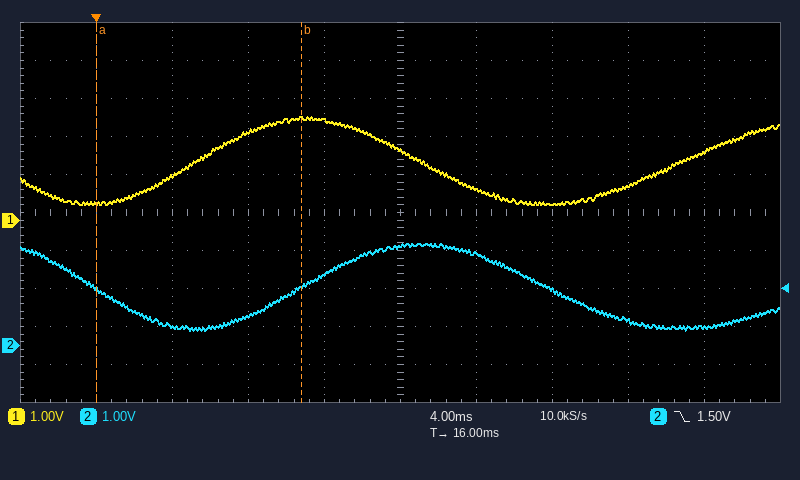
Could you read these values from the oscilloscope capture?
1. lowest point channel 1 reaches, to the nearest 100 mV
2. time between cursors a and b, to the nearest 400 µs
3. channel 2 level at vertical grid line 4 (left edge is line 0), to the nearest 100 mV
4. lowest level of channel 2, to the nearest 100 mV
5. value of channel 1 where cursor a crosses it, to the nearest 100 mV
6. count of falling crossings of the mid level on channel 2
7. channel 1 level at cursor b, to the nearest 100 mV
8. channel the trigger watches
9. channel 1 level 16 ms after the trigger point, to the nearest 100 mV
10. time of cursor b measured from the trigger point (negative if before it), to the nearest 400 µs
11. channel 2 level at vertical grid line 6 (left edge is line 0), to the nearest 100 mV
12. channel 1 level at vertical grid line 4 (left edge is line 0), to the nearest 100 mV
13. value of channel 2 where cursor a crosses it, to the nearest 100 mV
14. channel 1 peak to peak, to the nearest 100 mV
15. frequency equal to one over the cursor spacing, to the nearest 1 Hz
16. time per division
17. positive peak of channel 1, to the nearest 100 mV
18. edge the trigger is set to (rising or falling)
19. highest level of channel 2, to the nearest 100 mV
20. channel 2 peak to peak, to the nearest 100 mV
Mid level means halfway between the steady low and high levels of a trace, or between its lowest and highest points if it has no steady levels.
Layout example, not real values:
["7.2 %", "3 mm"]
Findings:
["400 mV", "10.8 ms", "1.9 V", "400 mV", "400 mV", "2", "2.7 V", "channel 2", "1.8 V", "+10.8 ms", "2.4 V", "2.6 V", "1.5 V", "2.3 V", "93 Hz", "4 ms", "2.7 V", "falling", "2.7 V", "2.3 V"]
